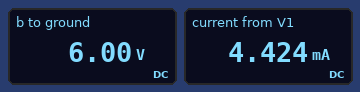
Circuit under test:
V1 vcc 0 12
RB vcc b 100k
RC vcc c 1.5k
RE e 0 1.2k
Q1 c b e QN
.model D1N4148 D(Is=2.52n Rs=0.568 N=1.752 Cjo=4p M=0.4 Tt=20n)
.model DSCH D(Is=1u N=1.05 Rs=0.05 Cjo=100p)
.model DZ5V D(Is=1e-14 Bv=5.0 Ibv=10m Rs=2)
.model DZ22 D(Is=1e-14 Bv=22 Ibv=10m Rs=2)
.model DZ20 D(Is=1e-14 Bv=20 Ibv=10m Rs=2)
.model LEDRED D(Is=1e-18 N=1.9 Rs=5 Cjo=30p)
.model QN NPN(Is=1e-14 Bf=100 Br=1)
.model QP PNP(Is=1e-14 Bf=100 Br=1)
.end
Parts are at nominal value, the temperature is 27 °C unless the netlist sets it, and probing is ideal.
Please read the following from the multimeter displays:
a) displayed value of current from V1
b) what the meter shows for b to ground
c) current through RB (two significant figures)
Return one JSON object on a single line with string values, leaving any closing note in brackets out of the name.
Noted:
{"displayed value of current from V1": "4.424 mA", "what the meter shows for b to ground": "6.00 V", "current through RB": "60 µA"}
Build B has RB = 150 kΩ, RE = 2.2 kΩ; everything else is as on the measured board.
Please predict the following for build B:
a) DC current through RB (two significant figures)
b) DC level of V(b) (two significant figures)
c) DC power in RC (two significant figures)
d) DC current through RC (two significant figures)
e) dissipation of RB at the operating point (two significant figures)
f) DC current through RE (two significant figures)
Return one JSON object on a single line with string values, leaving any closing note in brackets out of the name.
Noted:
{"DC current through RB": "30 µA", "DC level of V(b)": "7.4 V", "DC power in RC": "14 mW", "DC current through RC": "3.0 mA", "dissipation of RB at the operating point": "140 µW", "DC current through RE": "3.1 mA"}
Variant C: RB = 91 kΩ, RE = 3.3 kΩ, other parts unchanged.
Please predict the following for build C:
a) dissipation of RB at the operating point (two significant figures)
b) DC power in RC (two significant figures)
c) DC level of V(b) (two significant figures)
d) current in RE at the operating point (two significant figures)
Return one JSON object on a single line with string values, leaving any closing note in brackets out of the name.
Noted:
{"dissipation of RB at the operating point": "110 µW", "DC power in RC": "9.0 mW", "DC level of V(b)": "8.9 V", "current in RE at the operating point": "2.5 mA"}
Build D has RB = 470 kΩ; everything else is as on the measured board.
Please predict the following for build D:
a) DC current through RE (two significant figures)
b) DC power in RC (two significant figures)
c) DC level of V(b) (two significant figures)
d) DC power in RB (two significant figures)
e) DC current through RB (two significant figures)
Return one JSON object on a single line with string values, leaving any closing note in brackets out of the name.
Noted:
{"DC current through RE": "1.9 mA", "DC power in RC": "5.5 mW", "DC level of V(b)": "3.0 V", "DC power in RB": "170 µW", "DC current through RB": "19 µA"}
